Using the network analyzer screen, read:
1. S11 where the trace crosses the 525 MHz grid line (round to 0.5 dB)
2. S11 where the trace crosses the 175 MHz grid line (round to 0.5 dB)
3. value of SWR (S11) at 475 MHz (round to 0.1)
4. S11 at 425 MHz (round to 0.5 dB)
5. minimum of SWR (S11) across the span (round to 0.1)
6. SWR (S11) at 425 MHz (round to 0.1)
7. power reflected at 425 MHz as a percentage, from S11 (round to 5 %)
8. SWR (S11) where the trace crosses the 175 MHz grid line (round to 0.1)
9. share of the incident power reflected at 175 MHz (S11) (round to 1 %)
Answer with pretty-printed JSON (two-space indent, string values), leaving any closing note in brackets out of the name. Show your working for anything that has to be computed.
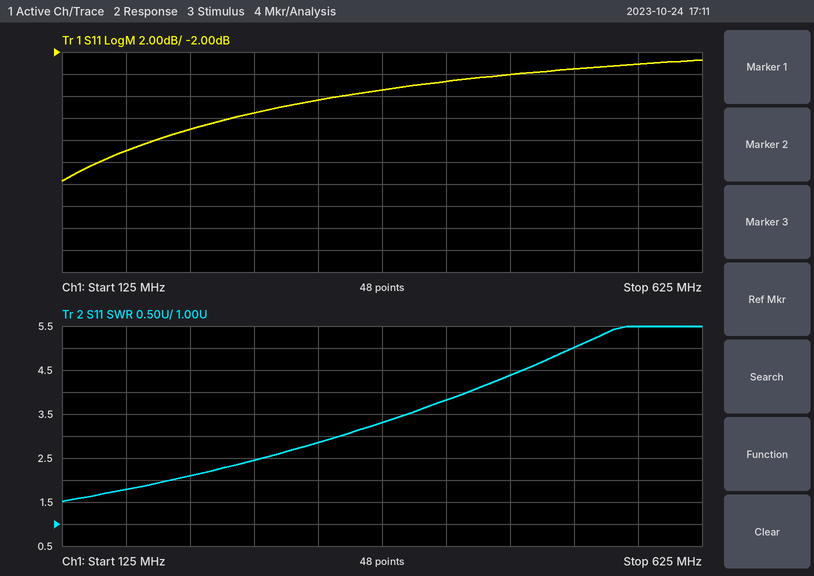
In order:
{
  "S11 where the trace crosses the 525 MHz grid line": "-3.5 dB",
  "S11 where the trace crosses the 175 MHz grid line": "-11.0 dB",
  "value of SWR (S11) at 475 MHz": "4.4",
  "S11 at 425 MHz": "-4.5 dB",
  "minimum of SWR (S11) across the span": "1.5",
  "SWR (S11) at 425 MHz": "3.8",
  "power reflected at 425 MHz as a percentage, from S11": "10^(-4.5/10) ≈ 35 %",
  "SWR (S11) where the trace crosses the 175 MHz grid line": "1.8",
  "share of the incident power reflected at 175 MHz (S11)": "10^(-11/10) ≈ 8 %"
}
